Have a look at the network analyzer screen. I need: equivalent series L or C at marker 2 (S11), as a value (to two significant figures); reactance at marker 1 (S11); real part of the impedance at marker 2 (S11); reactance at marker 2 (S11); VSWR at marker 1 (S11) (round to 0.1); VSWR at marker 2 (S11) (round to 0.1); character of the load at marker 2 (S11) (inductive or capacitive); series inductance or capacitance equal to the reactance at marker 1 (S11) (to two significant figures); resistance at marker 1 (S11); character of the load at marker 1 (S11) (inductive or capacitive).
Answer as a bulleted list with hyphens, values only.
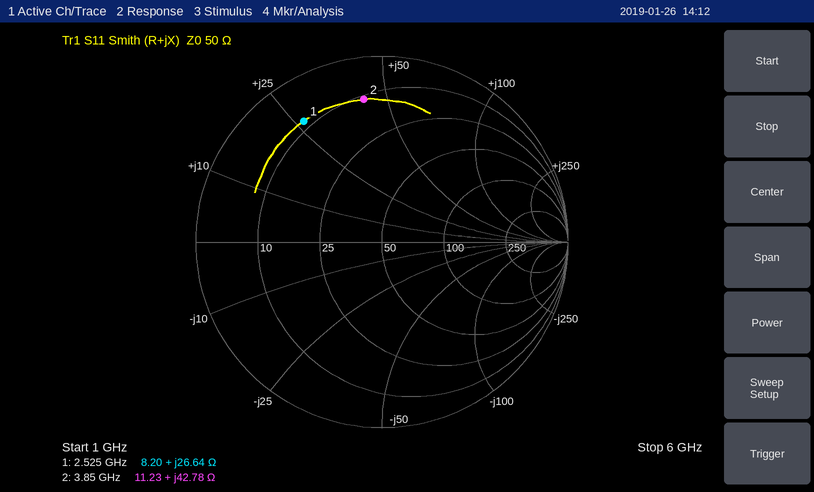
- 1.8 nH
- +26.64 Ω
- 11.23 Ω
- +42.78 Ω
- 7.9
- 7.8
- inductive
- 1.7 nH
- 8.20 Ω
- inductive
